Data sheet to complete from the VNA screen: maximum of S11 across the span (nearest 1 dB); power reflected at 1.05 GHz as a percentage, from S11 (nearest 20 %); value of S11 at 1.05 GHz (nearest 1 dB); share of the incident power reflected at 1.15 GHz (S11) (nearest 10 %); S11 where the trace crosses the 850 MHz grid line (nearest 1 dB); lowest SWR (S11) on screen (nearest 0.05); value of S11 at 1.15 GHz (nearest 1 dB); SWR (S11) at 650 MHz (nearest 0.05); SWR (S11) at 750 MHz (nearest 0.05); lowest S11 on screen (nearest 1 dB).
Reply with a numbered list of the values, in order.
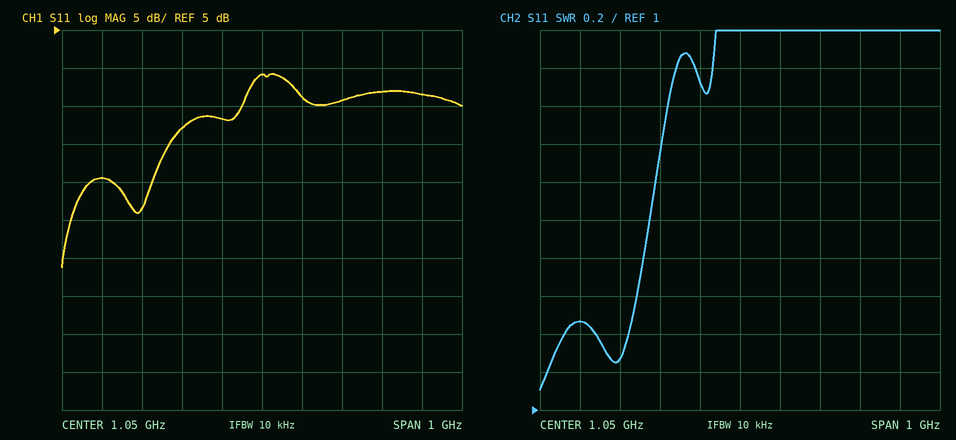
1. -1 dB
2. 80 %
3. -1 dB
4. 40 %
5. -8 dB
6. 1.10
7. -4 dB
8. 1.45
9. 1.25
10. -26 dB
